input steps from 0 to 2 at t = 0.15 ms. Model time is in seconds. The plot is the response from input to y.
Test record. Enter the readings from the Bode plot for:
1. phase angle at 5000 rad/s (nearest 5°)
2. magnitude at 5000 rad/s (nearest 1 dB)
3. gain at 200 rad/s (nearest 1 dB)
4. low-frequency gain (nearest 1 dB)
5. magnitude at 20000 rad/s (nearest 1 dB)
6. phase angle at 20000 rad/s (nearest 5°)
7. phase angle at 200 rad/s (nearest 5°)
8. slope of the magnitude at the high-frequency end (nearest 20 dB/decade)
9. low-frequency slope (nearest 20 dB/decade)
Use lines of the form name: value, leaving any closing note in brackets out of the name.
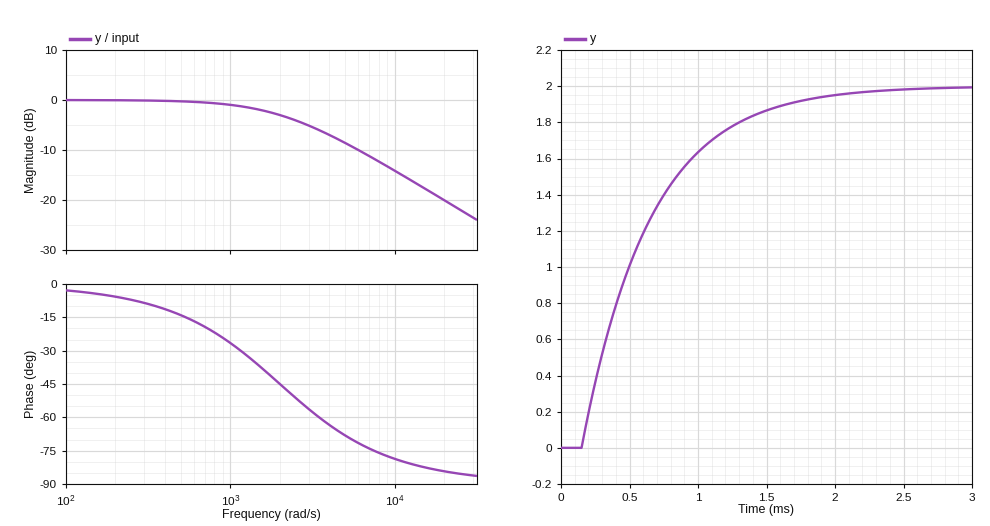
phase angle at 5000 rad/s: -70°
magnitude at 5000 rad/s: -9 dB
gain at 200 rad/s: 0 dB
low-frequency gain: 0 dB
magnitude at 20000 rad/s: -20 dB
phase angle at 20000 rad/s: -85°
phase angle at 200 rad/s: -5°
slope of the magnitude at the high-frequency end: -20 dB/decade
low-frequency slope: 0 dB/decade
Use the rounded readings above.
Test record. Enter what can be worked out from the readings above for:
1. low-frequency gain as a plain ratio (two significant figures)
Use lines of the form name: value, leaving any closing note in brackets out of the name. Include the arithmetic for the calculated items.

low-frequency gain as a plain ratio: 10^(0 / 20) = 1.0
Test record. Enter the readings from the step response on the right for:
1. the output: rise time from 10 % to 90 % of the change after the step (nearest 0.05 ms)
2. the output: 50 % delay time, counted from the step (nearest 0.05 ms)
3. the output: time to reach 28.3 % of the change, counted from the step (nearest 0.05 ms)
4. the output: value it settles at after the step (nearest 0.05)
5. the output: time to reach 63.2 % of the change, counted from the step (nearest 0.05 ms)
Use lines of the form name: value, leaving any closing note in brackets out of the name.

the output: rise time from 10 % to 90 % of the change after the step: 1.10 ms
the output: 50 % delay time, counted from the step: 0.35 ms
the output: time to reach 28.3 % of the change, counted from the step: 0.15 ms
the output: value it settles at after the step: 2.00
the output: time to reach 63.2 % of the change, counted from the step: 0.50 ms
